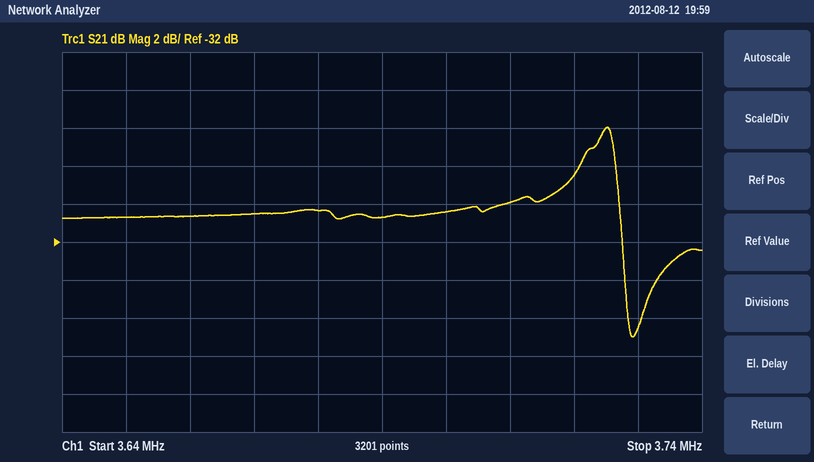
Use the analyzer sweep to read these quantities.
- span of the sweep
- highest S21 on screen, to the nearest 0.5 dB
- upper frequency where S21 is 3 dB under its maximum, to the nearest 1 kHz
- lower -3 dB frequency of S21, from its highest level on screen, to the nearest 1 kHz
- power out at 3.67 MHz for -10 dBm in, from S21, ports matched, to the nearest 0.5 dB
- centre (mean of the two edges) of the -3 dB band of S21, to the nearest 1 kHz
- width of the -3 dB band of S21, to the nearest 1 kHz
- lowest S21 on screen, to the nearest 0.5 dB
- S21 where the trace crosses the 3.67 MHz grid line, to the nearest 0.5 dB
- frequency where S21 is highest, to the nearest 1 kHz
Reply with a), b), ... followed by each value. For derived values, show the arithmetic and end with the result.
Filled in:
a) 100 kHz
b) -26.0 dB
c) 3.727 MHz
d) 3.719 MHz
e) -10 dBm + (-30.5 dB) = -40.5 dBm
f) 3.723 MHz
g) 3.727 MHz − 3.719 MHz = 8 kHz
h) -37.0 dB
i) -30.5 dB
j) 3.725 MHz
